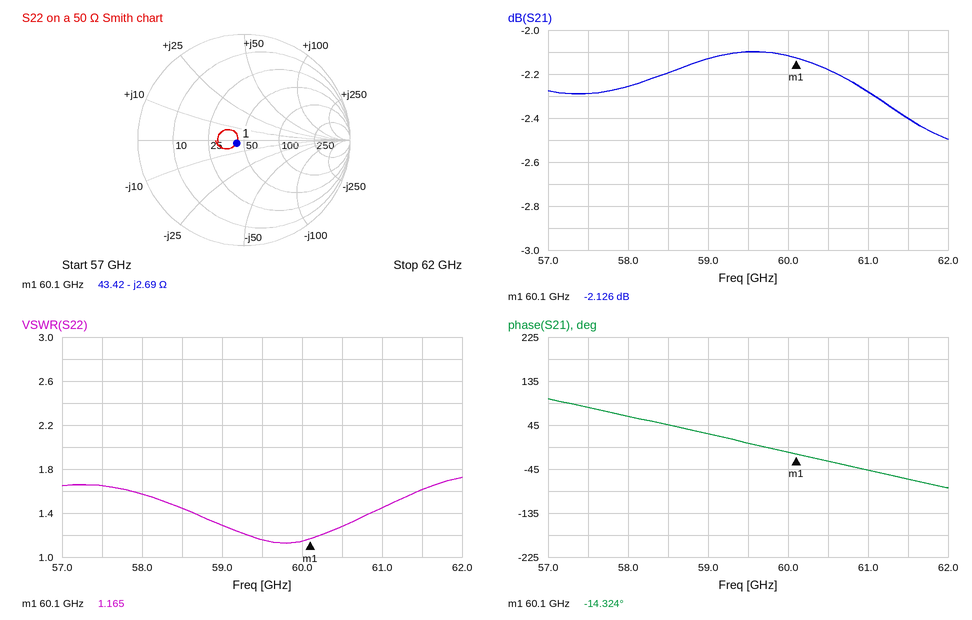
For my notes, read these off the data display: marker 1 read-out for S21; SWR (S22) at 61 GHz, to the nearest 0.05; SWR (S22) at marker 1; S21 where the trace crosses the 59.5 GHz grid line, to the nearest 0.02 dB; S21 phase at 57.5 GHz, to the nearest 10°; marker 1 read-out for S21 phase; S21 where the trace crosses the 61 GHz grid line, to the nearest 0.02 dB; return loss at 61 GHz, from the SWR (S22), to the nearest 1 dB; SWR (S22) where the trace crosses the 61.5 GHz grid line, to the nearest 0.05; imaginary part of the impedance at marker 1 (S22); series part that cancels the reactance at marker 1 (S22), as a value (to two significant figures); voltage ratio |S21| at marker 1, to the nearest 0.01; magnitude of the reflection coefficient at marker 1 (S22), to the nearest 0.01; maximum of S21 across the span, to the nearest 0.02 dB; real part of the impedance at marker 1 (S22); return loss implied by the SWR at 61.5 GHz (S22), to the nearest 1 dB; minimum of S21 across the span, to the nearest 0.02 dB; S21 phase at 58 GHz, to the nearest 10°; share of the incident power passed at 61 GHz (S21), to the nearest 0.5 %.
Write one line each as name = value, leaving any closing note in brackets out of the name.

marker 1 read-out for S21 = -2.126 dB
SWR (S22) at 61 GHz, to the nearest 0.05 = 1.45
SWR (S22) at marker 1 = 1.165
S21 where the trace crosses the 59.5 GHz grid line, to the nearest 0.02 dB = -2.10 dB
S21 phase at 57.5 GHz, to the nearest 10° = 80°
marker 1 read-out for S21 phase = -14.324°
S21 where the trace crosses the 61 GHz grid line, to the nearest 0.02 dB = -2.28 dB
return loss at 61 GHz, from the SWR (S22), to the nearest 1 dB = 15 dB
SWR (S22) where the trace crosses the 61.5 GHz grid line, to the nearest 0.05 = 1.60
imaginary part of the impedance at marker 1 = -2.69 Ω
series part that cancels the reactance at marker 1 (S22), as a value = 7.1 pH
voltage ratio |S21| at marker 1, to the nearest 0.01 = 0.78
magnitude of the reflection coefficient at marker 1 (S22), to the nearest 0.01 = 0.08
maximum of S21 across the span, to the nearest 0.02 dB = -2.10 dB
real part of the impedance at marker 1 = 43.42 Ω
return loss implied by the SWR at 61.5 GHz (S22), to the nearest 1 dB = 13 dB
minimum of S21 across the span, to the nearest 0.02 dB = -2.50 dB
S21 phase at 58 GHz, to the nearest 10° = 60°
share of the incident power passed at 61 GHz (S21), to the nearest 0.5 % = 59.0 %
